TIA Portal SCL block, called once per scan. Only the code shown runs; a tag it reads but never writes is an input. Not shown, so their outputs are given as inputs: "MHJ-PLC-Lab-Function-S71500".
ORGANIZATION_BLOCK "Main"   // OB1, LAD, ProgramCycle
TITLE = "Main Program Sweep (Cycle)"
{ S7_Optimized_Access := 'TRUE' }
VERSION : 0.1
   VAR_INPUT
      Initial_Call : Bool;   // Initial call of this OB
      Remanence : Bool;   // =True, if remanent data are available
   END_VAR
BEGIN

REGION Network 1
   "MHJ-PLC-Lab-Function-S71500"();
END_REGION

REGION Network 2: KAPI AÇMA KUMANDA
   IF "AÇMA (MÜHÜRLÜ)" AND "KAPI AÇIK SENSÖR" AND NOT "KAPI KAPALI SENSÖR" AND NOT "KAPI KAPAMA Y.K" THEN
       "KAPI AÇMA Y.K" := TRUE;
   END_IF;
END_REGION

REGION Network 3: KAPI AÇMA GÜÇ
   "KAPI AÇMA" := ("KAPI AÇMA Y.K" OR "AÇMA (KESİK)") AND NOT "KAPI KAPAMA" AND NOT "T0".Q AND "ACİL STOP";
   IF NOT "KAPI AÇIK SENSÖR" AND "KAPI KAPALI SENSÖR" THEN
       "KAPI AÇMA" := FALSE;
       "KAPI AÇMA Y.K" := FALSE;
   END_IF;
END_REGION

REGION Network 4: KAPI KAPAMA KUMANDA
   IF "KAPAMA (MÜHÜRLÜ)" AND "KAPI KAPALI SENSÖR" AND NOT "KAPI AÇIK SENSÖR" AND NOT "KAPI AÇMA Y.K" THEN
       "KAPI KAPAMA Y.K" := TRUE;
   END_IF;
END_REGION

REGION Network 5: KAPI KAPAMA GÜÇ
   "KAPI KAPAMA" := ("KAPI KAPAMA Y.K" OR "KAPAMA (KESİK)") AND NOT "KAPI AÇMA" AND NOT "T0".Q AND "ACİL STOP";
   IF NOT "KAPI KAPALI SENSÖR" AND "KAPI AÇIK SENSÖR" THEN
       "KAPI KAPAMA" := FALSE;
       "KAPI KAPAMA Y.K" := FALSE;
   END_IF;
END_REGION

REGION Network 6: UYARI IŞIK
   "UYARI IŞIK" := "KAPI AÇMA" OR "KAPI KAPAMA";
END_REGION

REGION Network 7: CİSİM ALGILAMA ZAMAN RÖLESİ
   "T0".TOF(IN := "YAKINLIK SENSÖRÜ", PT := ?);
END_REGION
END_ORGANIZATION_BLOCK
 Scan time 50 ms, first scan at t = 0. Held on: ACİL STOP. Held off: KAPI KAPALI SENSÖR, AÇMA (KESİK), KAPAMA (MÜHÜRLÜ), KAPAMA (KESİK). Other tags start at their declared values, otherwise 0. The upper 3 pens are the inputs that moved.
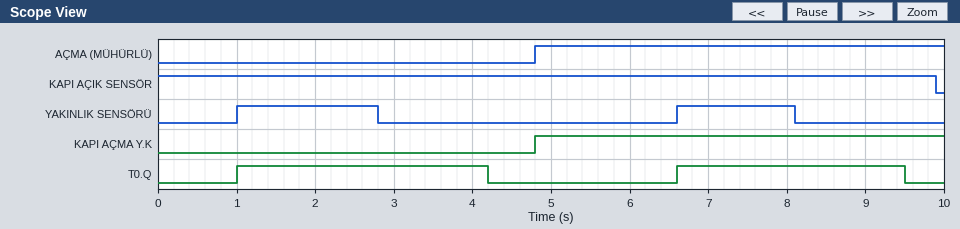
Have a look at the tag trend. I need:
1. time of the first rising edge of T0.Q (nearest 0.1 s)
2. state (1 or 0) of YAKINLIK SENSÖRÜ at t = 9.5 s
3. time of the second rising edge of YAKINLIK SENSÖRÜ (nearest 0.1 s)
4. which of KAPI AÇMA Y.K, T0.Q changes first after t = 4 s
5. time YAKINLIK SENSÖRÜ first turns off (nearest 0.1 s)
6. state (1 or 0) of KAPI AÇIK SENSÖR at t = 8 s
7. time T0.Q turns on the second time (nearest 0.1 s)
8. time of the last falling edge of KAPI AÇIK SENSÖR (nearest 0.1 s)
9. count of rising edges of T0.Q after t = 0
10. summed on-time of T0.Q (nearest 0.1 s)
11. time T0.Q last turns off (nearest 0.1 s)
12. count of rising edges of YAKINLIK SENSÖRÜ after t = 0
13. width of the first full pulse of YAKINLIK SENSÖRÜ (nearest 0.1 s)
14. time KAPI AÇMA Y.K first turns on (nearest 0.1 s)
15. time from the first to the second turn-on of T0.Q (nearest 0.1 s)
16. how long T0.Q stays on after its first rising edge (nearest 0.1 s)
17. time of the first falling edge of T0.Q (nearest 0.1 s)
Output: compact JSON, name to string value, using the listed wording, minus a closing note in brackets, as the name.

{"time of the first rising edge of T0.Q": "1.0 s", "state (1 or 0) of YAKINLIK SENSÖRÜ at t = 9.5 s": "0", "time of the second rising edge of YAKINLIK SENSÖRÜ": "6.6 s", "which of KAPI AÇMA Y.K, T0.Q changes first after t = 4 s": "T0.Q", "time YAKINLIK SENSÖRÜ first turns off": "2.8 s", "state (1 or 0) of KAPI AÇIK SENSÖR at t = 8 s": "1", "time T0.Q turns on the second time": "6.6 s", "time of the last falling edge of KAPI AÇIK SENSÖR": "9.9 s", "count of rising edges of T0.Q after t = 0": "2", "summed on-time of T0.Q": "6.1 s", "time T0.Q last turns off": "9.5 s", "count of rising edges of YAKINLIK SENSÖRÜ after t = 0": "2", "width of the first full pulse of YAKINLIK SENSÖRÜ": "1.8 s", "time KAPI AÇMA Y.K first turns on": "4.8 s", "time from the first to the second turn-on of T0.Q": "5.6 s", "how long T0.Q stays on after its first rising edge": "3.2 s", "time of the first falling edge of T0.Q": "4.2 s"}
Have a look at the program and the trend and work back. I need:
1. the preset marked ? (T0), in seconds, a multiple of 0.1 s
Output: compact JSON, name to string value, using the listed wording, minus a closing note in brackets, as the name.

{"the preset marked ? (T0), in seconds, a multiple of 0.1 s": "1.4 s"}
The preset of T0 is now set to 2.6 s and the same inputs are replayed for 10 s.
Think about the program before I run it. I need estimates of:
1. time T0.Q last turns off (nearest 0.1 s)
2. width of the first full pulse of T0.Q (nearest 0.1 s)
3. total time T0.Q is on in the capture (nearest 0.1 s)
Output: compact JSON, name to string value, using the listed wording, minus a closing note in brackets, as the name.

{"time T0.Q last turns off": "5.4 s", "width of the first full pulse of T0.Q": "4.4 s", "total time T0.Q is on in the capture": "7.8 s"}
